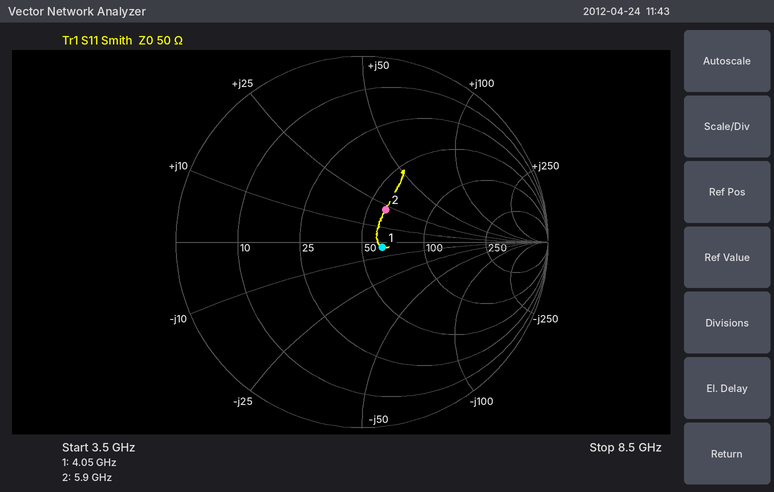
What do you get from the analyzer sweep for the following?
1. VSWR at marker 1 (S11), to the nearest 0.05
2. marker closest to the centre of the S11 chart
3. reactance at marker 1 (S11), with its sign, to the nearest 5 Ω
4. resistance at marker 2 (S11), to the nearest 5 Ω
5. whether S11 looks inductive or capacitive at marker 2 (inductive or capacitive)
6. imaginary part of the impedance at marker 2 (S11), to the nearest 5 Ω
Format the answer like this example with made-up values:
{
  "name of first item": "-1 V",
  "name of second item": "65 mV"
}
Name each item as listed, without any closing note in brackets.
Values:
{
  "VSWR at marker 1 (S11), to the nearest 0.05": "1.25",
  "marker closest to the centre of the S11 chart": "marker 1",
  "reactance at marker 1 (S11), with its sign, to the nearest 5 Ω": "-5 Ω",
  "resistance at marker 2 (S11), to the nearest 5 Ω": "60 Ω",
  "whether S11 looks inductive or capacitive at marker 2": "inductive",
  "imaginary part of the impedance at marker 2 (S11), to the nearest 5 Ω": "+20 Ω"
}
